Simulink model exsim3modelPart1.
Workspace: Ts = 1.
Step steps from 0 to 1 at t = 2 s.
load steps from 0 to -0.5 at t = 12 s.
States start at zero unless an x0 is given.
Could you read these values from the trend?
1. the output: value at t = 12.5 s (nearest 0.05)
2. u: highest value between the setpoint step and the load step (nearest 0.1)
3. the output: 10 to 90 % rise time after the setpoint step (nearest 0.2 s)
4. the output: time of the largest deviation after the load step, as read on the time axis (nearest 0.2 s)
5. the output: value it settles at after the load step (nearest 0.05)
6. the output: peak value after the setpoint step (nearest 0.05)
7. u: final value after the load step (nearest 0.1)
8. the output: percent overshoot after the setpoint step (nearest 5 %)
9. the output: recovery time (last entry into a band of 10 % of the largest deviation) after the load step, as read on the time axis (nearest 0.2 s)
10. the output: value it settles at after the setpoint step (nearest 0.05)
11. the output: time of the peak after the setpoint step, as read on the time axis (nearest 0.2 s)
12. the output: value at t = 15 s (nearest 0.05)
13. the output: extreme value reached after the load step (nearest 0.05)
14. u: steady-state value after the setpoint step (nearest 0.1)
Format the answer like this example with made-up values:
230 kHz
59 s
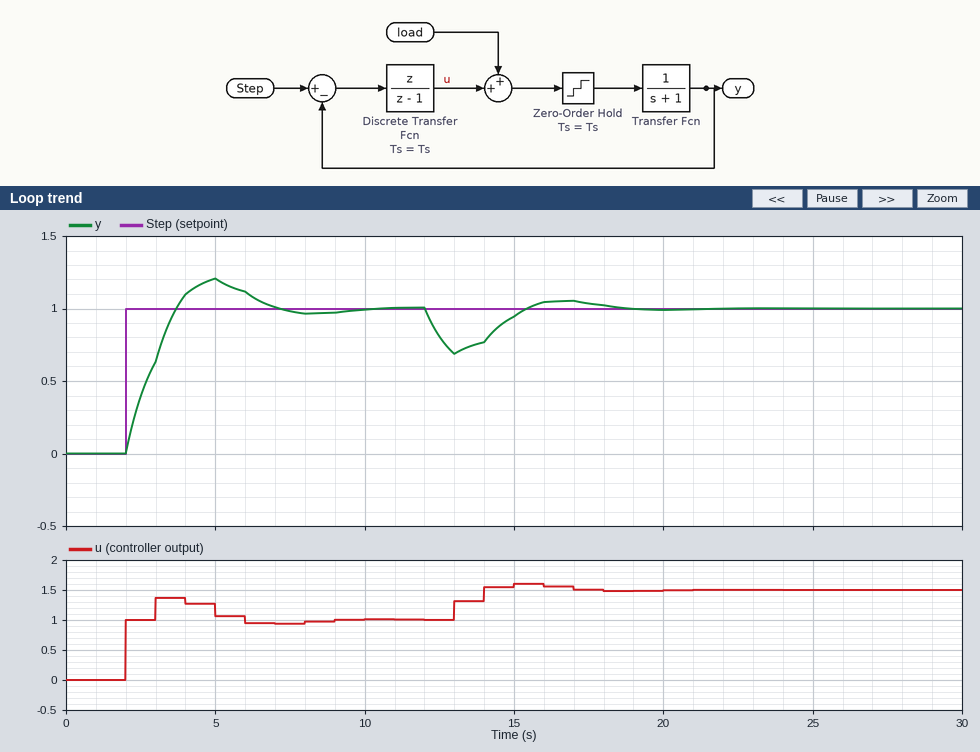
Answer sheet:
0.80
1.4
1.4 s
13.0 s
1.00
1.20
1.5
20 %
17.6 s
1.00
5.0 s
0.95
0.70
1.0
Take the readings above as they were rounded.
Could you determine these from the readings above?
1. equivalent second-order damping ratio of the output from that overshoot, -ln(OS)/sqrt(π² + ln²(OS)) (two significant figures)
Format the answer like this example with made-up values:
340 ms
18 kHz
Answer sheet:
0.46
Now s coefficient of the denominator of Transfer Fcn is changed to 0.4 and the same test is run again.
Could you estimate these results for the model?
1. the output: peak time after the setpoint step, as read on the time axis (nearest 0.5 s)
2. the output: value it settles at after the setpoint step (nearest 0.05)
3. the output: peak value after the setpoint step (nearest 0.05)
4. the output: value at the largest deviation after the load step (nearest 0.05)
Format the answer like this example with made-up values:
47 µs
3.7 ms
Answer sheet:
4.0 s
1.00
1.05
0.55
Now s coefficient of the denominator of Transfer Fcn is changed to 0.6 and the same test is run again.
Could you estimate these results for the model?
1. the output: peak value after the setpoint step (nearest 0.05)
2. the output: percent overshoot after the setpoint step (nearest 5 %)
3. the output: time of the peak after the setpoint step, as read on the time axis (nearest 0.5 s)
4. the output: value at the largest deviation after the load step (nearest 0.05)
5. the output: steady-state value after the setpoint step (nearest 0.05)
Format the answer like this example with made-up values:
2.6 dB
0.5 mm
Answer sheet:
1.10
10 %
4.0 s
0.60
1.00
